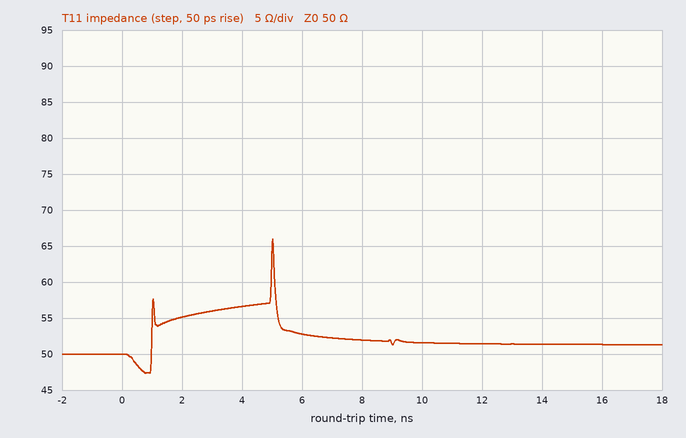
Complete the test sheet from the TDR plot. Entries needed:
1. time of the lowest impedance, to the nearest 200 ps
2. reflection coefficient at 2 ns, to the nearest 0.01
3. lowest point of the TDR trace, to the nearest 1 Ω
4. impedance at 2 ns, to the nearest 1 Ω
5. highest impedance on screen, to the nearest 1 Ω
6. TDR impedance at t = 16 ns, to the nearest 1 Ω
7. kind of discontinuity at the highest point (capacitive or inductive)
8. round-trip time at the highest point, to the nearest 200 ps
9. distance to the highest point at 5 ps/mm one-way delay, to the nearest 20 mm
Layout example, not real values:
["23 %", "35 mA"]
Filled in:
["800 ps", "+0.05", "47 Ω", "55 Ω", "66 Ω", "51 Ω", "inductive", "5.0 ns", "500 mm"]
